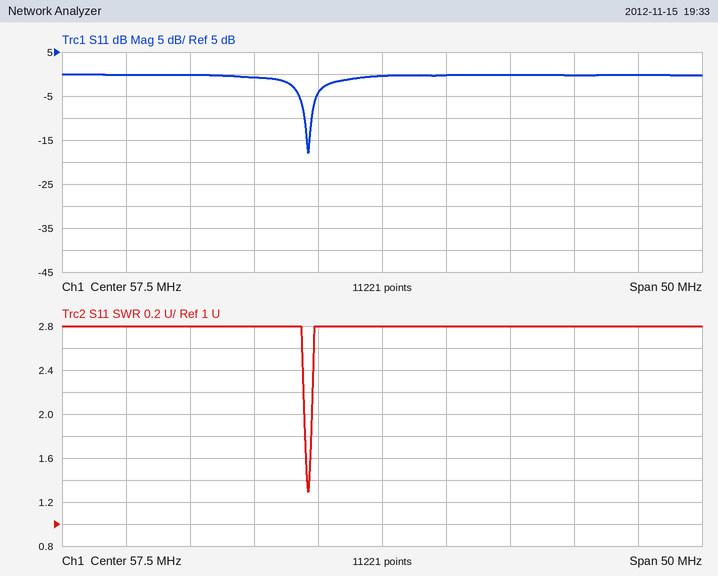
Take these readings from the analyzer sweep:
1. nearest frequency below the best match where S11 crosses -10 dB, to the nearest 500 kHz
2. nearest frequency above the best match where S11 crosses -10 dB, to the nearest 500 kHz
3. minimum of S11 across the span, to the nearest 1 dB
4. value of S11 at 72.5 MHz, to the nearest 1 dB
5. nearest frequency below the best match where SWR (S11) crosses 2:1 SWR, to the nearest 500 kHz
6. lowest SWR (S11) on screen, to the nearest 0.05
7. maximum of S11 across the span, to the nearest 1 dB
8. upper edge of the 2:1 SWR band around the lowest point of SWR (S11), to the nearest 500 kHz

51.5 MHz
52.0 MHz
-18 dB
0 dB
51.5 MHz
1.30
0 dB
52.0 MHz
